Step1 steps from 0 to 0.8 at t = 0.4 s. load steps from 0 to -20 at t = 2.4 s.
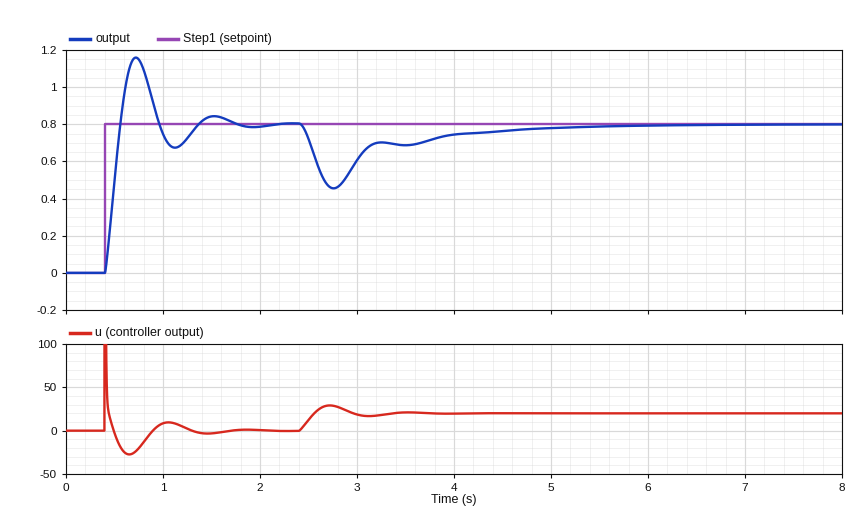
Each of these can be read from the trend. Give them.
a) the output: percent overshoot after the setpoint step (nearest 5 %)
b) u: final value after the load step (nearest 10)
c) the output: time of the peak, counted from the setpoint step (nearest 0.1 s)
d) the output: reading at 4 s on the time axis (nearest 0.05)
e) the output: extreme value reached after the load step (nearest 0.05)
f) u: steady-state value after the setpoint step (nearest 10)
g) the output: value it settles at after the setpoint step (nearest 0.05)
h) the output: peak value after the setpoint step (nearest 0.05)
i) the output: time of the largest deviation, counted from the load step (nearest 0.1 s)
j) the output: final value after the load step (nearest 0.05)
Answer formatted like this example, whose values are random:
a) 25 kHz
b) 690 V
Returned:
a) 45 %
b) 20
c) 0.3 s
d) 0.75
e) 0.45
f) 0
g) 0.80
h) 1.15
i) 0.4 s
j) 0.80
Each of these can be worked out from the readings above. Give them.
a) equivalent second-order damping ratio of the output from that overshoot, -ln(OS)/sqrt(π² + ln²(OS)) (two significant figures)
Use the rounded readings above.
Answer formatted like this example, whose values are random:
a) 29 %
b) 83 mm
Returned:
a) 0.25
